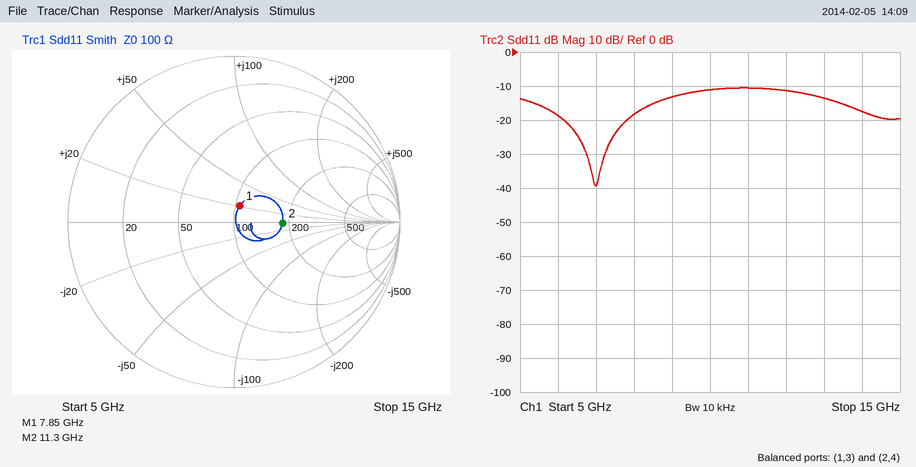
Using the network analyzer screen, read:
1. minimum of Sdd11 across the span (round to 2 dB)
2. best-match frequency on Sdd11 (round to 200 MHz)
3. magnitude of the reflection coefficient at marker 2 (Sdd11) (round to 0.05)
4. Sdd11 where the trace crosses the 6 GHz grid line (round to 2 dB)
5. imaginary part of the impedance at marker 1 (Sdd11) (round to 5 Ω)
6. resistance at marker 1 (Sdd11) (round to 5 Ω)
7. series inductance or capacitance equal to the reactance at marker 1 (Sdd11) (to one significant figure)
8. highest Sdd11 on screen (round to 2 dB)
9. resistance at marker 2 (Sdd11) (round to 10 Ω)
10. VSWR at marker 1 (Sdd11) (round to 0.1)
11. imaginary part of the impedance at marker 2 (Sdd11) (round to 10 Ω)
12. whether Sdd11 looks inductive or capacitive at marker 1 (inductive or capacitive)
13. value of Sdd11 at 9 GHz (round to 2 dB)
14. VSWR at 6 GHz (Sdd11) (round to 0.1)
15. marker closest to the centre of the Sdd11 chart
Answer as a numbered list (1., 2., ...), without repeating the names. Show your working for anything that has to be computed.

1. -40 dB
2. 7.0 GHz
3. 0.30
4. -18 dB
5. +20 Ω
6. 105 Ω
7. L = 20 Ω/(2π × 7.85 GHz) ≈ 405 pH, so 400 pH to one significant figure
8. -10 dB
9. 180 Ω
10. 1.2
11. 0 Ω
12. inductive
13. -14 dB
14. |Γ| = 10^(-18/20) = 0.1259; VSWR = (1 + 0.1259)/(1 − 0.1259) ≈ 1.3
15. marker 1
